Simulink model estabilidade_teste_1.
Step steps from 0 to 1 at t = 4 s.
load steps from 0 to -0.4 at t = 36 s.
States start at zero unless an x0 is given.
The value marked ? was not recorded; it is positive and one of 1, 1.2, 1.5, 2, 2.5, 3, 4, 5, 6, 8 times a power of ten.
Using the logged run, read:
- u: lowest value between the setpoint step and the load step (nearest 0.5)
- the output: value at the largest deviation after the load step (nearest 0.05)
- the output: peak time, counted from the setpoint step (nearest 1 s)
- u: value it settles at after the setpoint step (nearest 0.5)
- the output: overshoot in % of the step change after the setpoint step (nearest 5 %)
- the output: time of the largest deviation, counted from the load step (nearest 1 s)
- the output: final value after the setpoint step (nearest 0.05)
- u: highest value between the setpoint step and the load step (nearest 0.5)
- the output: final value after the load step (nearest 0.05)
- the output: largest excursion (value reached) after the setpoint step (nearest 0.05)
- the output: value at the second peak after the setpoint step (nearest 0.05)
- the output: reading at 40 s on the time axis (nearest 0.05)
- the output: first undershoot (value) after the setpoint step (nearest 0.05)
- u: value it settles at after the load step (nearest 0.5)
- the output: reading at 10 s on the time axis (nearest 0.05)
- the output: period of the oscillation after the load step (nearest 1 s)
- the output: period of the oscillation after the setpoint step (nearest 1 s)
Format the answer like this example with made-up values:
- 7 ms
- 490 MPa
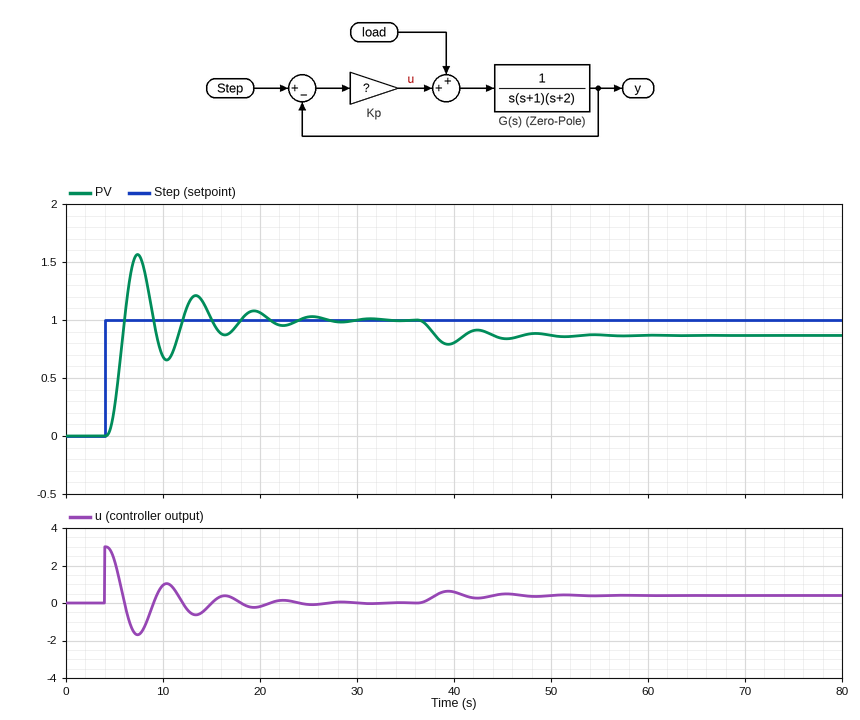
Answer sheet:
- -1.5
- 0.80
- 3 s
- 0.0
- 55 %
- 3 s
- 1.00
- 3.0
- 0.85
- 1.55
- 1.20
- 0.80
- 0.65
- 0.5
- 0.70
- 6 s
- 6 s
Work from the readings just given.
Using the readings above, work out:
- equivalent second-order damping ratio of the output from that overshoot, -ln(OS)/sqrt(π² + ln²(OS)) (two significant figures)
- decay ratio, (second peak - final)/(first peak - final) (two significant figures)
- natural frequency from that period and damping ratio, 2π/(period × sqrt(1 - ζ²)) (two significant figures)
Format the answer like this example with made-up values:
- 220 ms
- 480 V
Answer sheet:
- 0.19
- 0.36
- 1.1 rad/s
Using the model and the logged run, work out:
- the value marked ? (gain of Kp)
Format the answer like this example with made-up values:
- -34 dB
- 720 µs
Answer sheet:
- 3
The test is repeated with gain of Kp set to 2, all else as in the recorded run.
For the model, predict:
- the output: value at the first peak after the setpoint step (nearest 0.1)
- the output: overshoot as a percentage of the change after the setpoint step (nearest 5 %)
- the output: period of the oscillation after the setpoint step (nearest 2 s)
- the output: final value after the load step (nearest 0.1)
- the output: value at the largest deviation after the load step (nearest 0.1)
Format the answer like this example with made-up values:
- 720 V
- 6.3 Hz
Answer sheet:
- 1.4
- 40 %
- 8 s
- 0.8
- 0.7
